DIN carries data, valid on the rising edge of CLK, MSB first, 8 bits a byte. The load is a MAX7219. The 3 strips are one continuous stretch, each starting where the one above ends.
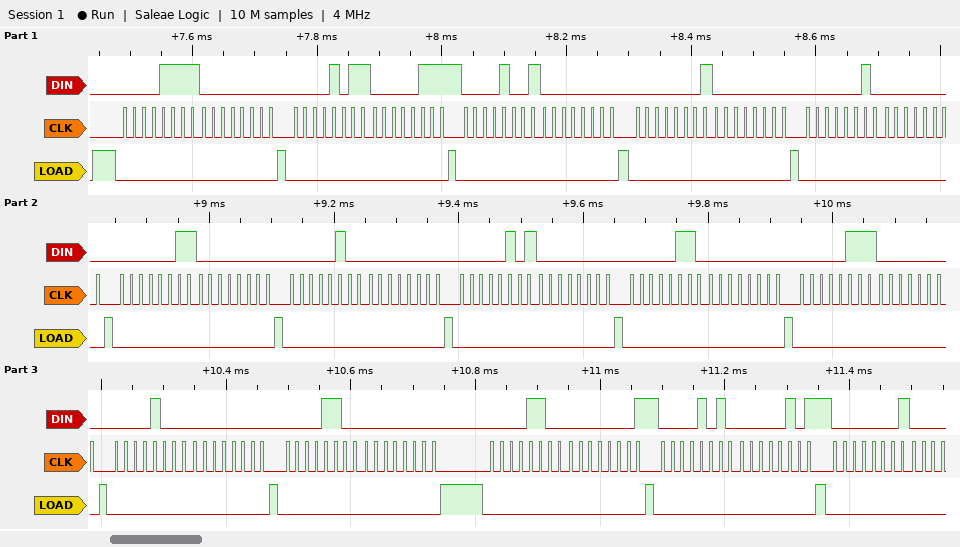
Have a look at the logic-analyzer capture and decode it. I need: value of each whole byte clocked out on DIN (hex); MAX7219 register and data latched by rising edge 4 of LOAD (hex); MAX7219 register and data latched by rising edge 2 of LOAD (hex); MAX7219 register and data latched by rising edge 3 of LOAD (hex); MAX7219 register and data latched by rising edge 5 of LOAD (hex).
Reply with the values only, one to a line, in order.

0F 00 0B 07 09 00 01 00 02 00 03 00 04 00 05 00 06 00 07 00 08 00 0C 00 0C 01 0A 05 01
register 0x9, data 0x00
register 0xF, data 0x00
register 0xB, data 0x07
register 0x1, data 0x00
